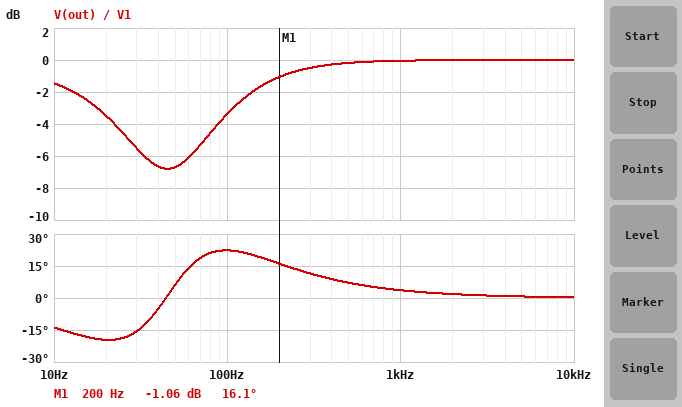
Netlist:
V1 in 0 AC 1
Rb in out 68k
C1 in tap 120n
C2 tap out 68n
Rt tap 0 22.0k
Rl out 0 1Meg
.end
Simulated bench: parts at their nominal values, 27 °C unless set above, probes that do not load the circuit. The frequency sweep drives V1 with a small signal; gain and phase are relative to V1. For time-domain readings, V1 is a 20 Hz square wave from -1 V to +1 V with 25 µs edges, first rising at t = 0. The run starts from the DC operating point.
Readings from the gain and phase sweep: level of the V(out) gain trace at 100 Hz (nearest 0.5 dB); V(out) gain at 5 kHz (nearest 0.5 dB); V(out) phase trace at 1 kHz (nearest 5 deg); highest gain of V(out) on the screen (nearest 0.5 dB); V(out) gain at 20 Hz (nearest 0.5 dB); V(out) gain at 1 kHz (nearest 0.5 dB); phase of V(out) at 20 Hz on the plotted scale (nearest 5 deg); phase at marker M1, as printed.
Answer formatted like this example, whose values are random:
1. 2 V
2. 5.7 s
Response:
1. -3.5 dB
2. 0 dB
3. 5 deg
4. 0 dB
5. -3.5 dB
6. 0 dB
7. -20 deg
8. 16.1 deg
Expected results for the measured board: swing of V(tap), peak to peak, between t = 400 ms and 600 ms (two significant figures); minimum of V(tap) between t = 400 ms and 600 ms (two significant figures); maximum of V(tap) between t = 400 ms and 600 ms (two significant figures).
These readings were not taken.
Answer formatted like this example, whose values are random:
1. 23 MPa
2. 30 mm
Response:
1. 3.9 V
2. -2.0 V
3. 2.0 V
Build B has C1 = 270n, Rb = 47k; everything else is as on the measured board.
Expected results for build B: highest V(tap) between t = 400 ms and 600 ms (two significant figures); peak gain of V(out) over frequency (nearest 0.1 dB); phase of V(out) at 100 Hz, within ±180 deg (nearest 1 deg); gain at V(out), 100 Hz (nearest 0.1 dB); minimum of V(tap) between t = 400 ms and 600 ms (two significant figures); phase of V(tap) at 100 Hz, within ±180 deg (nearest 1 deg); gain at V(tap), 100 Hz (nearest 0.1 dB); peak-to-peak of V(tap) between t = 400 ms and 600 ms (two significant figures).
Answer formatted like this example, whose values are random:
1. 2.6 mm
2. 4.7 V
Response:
1. 1.9 V
2. 0 dB
3. 11 deg
4. -1.4 dB
5. -1.9 V
6. 14 deg
7. -0.5 dB
8. 3.8 V
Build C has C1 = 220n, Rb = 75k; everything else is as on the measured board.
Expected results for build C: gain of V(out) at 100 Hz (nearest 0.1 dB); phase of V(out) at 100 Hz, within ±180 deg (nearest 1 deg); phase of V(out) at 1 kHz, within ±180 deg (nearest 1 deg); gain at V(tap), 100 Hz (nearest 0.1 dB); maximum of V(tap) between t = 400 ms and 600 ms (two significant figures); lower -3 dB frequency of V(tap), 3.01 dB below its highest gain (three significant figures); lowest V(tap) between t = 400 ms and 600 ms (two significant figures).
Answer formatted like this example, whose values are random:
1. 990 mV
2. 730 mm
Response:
1. -1.5 dB
2. 16 deg
3. 2 deg
4. -0.7 dB
5. 1.9 V
6. 32.9 Hz
7. -1.9 V
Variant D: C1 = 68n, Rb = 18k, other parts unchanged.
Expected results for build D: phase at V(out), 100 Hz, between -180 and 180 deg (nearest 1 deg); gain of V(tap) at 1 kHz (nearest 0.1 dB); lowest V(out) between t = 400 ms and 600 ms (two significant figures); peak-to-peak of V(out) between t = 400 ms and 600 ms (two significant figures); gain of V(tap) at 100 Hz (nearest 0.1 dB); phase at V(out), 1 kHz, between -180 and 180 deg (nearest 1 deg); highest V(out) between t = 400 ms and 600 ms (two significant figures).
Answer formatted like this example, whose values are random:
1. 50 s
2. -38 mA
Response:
1. -2 deg
2. -0.2 dB
3. -1.0 V
4. 2.0 V
5. -2.5 dB
6. 6 deg
7. 1.0 V
